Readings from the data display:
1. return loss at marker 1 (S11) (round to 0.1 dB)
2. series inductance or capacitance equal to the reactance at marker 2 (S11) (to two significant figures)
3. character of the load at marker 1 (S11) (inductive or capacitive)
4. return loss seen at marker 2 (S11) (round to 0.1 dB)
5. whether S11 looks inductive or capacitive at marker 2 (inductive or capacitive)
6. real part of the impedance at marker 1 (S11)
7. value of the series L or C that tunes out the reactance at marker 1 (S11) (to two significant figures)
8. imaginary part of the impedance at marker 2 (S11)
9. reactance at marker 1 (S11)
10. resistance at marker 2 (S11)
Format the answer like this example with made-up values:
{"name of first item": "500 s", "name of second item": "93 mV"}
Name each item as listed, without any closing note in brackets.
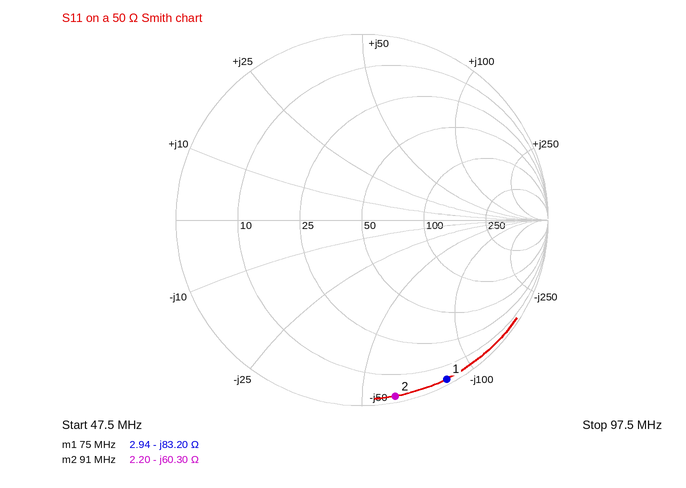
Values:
{"return loss at marker 1 (S11)": "0.3 dB", "series inductance or capacitance equal to the reactance at marker 2 (S11)": "29 pF", "character of the load at marker 1 (S11)": "capacitive", "return loss seen at marker 2 (S11)": "0.3 dB", "whether S11 looks inductive or capacitive at marker 2": "capacitive", "real part of the impedance at marker 1": "2.94 Ω", "value of the series L or C that tunes out the reactance at marker 1 (S11)": "180 nH", "imaginary part of the impedance at marker 2": "-60.30 Ω", "reactance at marker 1": "-83.20 Ω", "resistance at marker 2": "2.20 Ω"}
